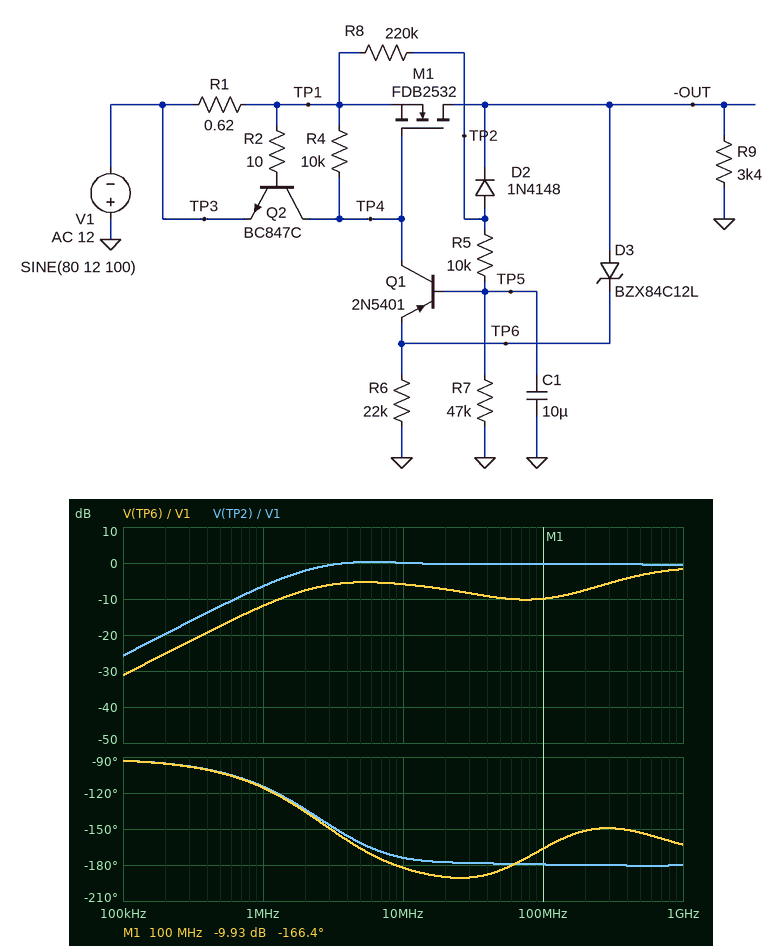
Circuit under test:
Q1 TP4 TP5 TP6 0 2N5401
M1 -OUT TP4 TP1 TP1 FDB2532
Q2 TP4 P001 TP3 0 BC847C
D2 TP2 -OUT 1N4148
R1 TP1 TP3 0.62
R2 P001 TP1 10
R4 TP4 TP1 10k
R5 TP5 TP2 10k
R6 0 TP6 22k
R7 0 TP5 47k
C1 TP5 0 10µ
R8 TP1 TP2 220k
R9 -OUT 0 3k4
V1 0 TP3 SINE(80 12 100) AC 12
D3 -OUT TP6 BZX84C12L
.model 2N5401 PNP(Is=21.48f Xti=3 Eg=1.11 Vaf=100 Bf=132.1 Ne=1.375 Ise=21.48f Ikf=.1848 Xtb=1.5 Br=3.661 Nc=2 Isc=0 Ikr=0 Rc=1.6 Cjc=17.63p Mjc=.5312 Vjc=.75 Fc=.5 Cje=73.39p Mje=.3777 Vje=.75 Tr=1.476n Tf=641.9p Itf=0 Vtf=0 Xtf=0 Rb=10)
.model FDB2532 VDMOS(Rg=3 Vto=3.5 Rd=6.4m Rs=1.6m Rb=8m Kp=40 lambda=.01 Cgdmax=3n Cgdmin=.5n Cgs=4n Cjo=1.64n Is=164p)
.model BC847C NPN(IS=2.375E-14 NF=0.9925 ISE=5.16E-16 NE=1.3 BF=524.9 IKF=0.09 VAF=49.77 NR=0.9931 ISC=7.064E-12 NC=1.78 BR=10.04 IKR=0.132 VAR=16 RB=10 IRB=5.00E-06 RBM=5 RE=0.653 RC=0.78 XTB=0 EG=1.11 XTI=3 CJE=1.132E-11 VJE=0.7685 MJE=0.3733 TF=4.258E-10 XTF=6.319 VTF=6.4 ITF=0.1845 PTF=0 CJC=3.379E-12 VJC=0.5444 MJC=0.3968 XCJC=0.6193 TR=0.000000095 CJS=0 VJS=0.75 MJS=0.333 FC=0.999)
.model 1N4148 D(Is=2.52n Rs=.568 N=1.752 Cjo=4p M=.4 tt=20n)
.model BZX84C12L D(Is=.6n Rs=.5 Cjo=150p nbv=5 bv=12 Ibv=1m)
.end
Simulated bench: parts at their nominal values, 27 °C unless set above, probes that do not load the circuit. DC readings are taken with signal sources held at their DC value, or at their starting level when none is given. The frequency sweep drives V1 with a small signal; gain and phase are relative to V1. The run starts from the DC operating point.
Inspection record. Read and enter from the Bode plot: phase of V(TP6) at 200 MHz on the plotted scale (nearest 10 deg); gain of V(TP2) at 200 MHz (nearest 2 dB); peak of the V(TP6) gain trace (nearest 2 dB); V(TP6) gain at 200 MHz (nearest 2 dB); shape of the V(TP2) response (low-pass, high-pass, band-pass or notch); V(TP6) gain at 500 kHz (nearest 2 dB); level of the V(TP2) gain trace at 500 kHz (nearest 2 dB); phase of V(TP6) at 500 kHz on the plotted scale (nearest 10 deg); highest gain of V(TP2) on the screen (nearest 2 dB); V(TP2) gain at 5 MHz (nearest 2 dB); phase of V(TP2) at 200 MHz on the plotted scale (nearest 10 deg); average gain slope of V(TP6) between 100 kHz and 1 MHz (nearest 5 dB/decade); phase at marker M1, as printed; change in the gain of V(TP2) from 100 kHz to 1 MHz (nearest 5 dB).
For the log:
-150 deg
0 dB
-2 dB
-8 dB
high-pass
-18 dB
-12 dB
-100 deg
0 dB
0 dB
-180 deg
20 dB/decade
-166.4 deg
20 dB
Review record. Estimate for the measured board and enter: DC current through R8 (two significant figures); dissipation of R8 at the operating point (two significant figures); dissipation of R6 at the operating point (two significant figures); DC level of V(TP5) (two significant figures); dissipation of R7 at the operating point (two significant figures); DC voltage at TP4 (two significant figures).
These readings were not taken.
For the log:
82 µA
1.5 mW
120 mW
-51 V
56 mW
-77 V
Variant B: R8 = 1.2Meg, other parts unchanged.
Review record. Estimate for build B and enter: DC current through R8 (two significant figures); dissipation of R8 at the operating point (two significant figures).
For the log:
15 µA
270 µW
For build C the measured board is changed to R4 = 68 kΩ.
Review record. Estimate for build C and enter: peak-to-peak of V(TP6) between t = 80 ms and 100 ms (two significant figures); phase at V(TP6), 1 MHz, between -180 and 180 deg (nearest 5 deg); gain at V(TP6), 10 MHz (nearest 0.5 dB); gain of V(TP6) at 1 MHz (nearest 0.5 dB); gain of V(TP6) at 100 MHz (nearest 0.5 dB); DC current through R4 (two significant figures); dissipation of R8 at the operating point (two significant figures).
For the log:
7.1 mV
-155 deg
-2.5 dB
-1.5 dB
-9.5 dB
50 µA
1.4 mW
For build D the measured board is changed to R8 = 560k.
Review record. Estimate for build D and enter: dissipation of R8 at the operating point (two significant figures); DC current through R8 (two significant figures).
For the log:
580 µW
32 µA
